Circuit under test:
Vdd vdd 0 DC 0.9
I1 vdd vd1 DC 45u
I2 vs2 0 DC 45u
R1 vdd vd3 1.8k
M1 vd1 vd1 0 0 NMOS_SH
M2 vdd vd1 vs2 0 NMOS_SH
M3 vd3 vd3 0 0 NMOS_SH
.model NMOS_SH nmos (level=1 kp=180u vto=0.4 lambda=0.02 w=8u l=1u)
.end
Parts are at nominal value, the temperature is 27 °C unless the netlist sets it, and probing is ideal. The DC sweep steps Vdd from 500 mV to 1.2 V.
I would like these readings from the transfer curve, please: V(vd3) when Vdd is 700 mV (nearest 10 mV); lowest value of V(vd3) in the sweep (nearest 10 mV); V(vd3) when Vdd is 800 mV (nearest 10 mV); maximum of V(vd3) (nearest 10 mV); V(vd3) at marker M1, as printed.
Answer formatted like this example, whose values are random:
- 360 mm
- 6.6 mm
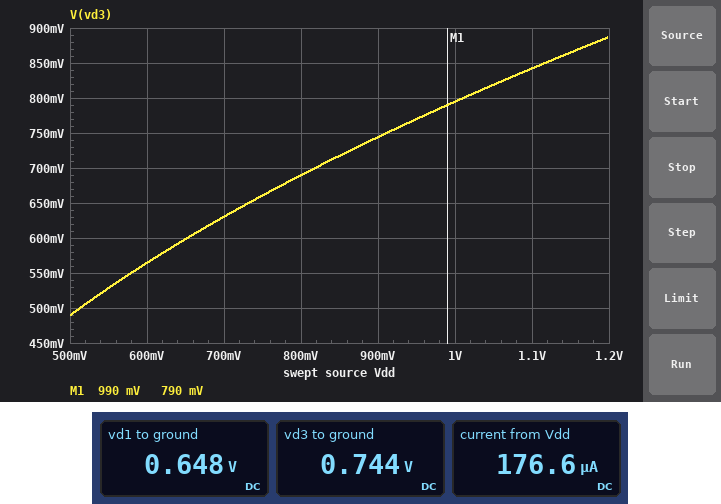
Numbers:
- 630 mV
- 490 mV
- 690 mV
- 890 mV
- 790 mV
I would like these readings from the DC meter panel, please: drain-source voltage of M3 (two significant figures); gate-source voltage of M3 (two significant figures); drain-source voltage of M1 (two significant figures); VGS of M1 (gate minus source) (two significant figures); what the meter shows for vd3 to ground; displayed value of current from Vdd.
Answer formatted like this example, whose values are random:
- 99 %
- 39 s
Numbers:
- 740 mV
- 740 mV
- 650 mV
- 650 mV
- 0.744 V
- 176.6 µA
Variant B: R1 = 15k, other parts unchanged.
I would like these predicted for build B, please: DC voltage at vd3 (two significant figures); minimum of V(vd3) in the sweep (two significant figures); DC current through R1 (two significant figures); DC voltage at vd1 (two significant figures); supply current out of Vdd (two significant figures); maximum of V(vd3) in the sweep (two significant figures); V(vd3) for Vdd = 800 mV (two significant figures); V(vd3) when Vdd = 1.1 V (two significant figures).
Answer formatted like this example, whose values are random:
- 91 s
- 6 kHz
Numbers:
- 570 mV
- 460 mV
- 22 µA
- 650 mV
- 110 µA
- 630 mV
- 550 mV
- 610 mV
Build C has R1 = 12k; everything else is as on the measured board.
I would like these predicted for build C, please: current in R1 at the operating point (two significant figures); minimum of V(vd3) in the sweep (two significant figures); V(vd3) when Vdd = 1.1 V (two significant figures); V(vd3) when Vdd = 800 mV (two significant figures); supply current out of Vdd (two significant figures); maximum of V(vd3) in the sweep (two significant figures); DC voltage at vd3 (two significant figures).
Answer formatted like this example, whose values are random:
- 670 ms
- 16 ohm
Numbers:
- 26 µA
- 460 mV
- 630 mV
- 560 mV
- 120 µA
- 650 mV
- 590 mV
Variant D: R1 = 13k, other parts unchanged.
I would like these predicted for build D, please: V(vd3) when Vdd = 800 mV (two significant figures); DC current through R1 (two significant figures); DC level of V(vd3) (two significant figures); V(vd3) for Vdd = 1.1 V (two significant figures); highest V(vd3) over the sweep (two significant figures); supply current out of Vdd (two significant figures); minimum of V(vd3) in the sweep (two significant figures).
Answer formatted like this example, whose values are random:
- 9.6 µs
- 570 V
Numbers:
- 560 mV
- 24 µA
- 580 mV
- 620 mV
- 640 mV
- 110 µA
- 460 mV
